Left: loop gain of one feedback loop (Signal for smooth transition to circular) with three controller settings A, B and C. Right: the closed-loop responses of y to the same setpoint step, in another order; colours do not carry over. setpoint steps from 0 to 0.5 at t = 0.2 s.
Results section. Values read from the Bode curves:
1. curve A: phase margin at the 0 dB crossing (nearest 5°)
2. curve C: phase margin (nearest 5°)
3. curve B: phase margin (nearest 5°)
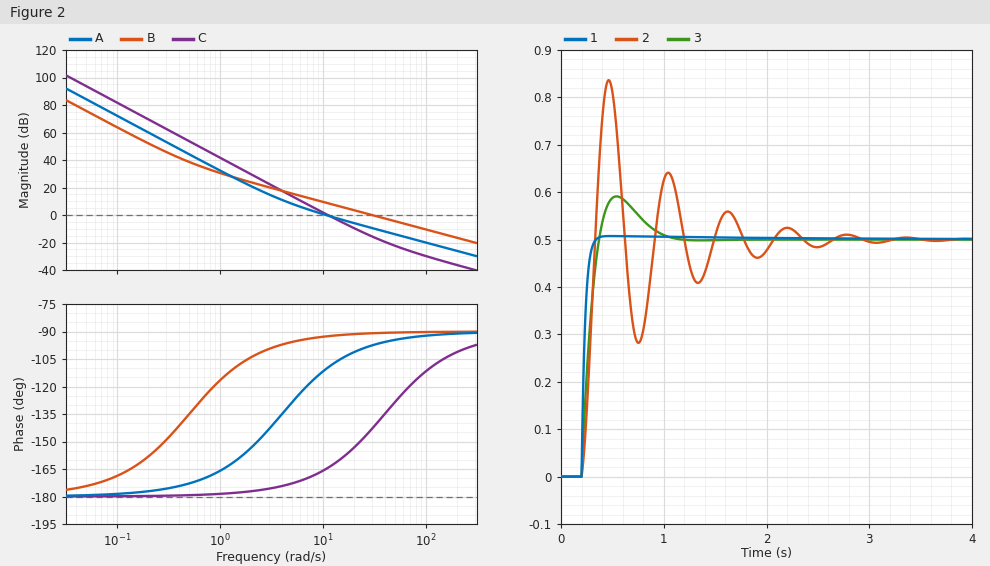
70°
15°
90°
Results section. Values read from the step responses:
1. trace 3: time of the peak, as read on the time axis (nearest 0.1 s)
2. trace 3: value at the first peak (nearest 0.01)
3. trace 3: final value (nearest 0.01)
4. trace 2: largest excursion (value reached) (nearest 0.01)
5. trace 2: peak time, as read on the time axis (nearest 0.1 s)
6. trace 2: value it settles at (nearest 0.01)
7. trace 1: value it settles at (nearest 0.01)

0.5 s
0.59
0.50
0.84
0.5 s
0.50
0.50
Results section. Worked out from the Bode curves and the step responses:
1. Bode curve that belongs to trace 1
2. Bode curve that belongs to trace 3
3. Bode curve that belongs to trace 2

B
A
C
